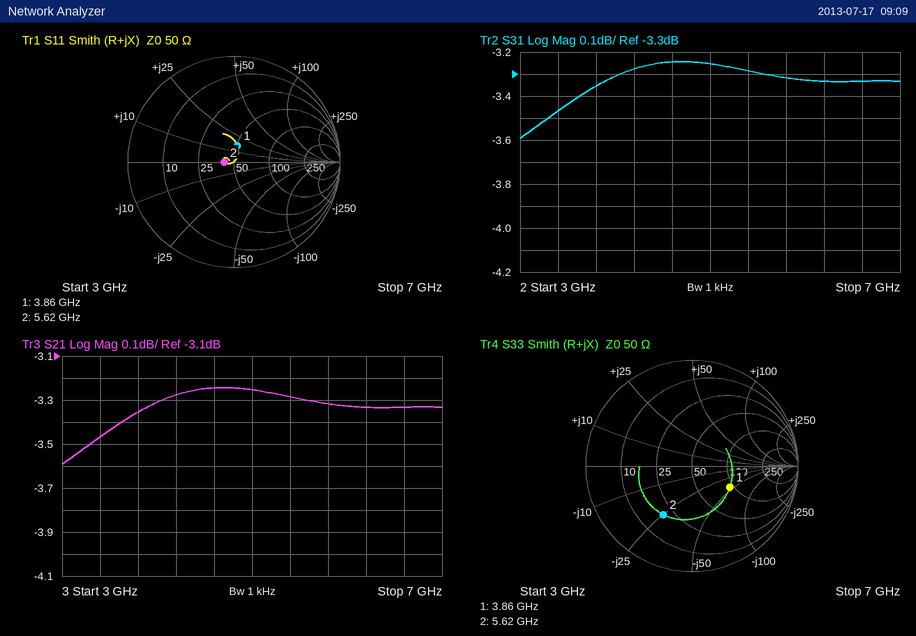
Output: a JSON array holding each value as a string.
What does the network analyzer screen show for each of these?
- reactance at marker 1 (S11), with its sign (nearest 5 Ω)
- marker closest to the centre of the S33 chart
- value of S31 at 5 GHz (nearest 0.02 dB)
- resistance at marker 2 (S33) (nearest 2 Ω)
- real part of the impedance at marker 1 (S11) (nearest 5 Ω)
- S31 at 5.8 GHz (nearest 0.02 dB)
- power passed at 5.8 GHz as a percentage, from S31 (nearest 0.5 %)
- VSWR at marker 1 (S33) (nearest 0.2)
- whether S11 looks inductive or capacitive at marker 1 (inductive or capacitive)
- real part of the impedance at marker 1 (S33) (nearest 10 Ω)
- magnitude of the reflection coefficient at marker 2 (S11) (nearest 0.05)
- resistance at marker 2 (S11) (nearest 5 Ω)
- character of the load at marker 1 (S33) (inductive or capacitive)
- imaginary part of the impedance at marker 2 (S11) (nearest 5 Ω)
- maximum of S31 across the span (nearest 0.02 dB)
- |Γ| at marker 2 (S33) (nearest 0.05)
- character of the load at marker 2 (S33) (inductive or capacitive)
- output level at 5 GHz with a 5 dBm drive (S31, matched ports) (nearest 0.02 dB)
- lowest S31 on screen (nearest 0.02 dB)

["+15 Ω", "marker 1", "-3.26 dB", "20 Ω", "50 Ω", "-3.32 dB", "46.5 %", "2.4", "inductive", "90 Ω", "0.10", "40 Ω", "capacitive", "0 Ω", "-3.24 dB", "0.55", "capacitive", "1.74 dBm", "-3.60 dB"]
